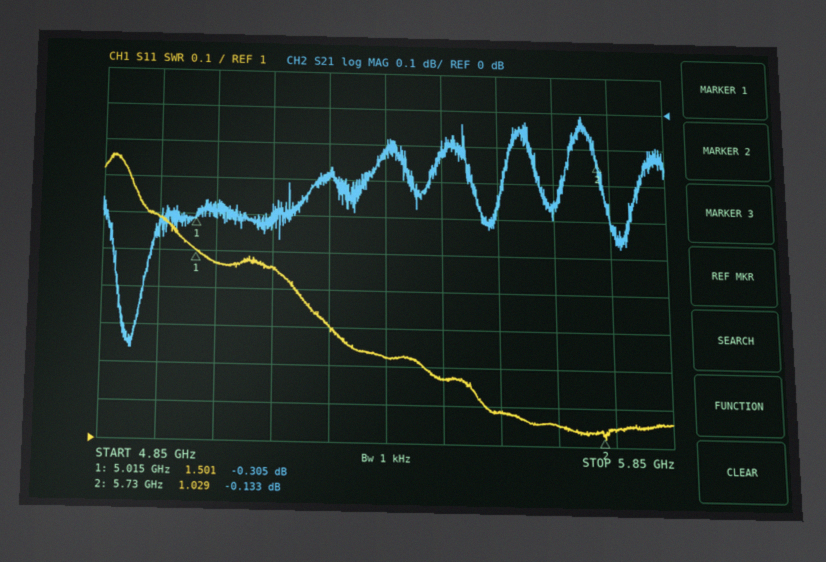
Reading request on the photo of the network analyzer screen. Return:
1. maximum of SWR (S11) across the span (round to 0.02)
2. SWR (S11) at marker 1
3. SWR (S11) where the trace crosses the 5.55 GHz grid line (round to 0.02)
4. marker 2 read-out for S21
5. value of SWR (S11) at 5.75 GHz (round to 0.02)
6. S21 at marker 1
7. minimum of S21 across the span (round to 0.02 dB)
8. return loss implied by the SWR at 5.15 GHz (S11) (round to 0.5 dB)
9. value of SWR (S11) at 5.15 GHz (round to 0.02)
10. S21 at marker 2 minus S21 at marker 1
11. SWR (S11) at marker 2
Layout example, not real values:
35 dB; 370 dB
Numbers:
1.76; 1.501; 1.08; -0.133 dB; 1.04; -0.305 dB; -0.66 dB; 14.5 dB; 1.46; 0.172 dB; 1.029
